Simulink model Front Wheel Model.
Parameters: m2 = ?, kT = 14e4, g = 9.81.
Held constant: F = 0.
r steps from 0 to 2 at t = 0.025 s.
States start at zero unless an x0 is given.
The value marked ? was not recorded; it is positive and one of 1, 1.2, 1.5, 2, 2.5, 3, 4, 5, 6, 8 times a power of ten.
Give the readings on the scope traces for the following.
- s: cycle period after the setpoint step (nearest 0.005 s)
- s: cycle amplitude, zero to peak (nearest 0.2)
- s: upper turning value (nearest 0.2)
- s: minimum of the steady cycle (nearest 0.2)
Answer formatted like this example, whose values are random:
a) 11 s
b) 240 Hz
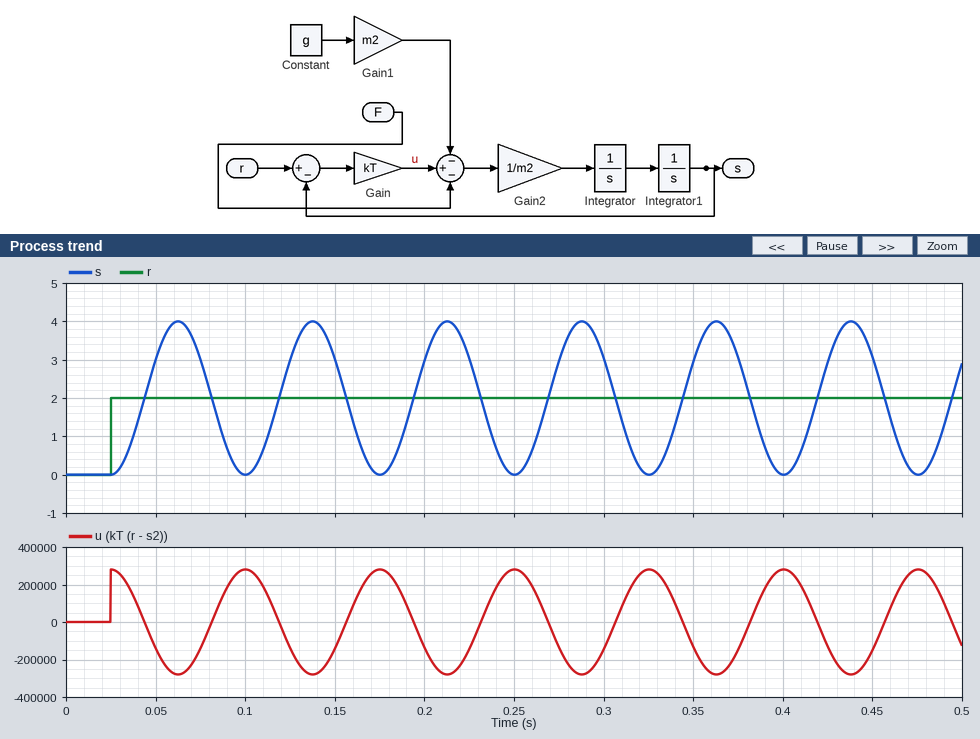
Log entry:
a) 0.075 s
b) 2.0
c) 4.0
d) 0.0
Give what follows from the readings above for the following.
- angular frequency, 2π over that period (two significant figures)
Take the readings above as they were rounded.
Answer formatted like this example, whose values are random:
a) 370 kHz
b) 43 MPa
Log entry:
a) 84 rad/s
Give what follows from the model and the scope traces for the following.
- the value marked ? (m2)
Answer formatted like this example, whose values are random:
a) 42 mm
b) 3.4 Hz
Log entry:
a) 20
